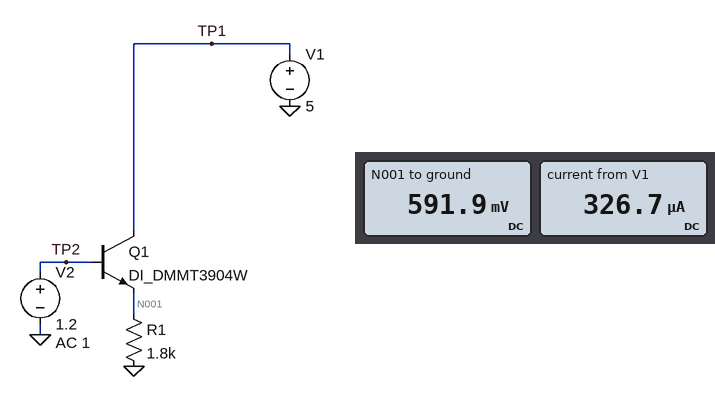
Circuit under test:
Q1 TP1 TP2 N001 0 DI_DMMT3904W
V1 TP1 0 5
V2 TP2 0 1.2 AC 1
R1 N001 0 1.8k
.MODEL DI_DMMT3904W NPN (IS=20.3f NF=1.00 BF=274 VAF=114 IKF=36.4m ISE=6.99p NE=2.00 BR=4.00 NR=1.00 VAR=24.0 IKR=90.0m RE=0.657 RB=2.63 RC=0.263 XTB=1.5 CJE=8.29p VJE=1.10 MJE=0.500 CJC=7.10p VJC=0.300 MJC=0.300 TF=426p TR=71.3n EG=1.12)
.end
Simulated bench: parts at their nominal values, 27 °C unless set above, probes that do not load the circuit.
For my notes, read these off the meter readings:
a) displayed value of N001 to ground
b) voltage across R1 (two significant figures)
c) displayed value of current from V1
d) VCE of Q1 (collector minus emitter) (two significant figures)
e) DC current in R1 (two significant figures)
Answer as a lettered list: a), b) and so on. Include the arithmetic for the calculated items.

a) 591.9 mV
b) 591.9 mV = 590 mV
c) 326.7 µA
d) 5 V - 591.9 mV = 4.4 V
e) (591.9 mV) / 1.8 kΩ = 330 µA
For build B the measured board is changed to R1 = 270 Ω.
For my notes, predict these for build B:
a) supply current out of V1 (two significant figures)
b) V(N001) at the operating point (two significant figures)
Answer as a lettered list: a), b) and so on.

a) 2.0 mA
b) 540 mV
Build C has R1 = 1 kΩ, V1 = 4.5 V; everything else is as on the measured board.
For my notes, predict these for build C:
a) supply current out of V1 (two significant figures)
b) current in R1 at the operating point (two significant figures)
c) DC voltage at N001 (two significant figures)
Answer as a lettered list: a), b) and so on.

a) 570 µA
b) 580 µA
c) 580 mV
